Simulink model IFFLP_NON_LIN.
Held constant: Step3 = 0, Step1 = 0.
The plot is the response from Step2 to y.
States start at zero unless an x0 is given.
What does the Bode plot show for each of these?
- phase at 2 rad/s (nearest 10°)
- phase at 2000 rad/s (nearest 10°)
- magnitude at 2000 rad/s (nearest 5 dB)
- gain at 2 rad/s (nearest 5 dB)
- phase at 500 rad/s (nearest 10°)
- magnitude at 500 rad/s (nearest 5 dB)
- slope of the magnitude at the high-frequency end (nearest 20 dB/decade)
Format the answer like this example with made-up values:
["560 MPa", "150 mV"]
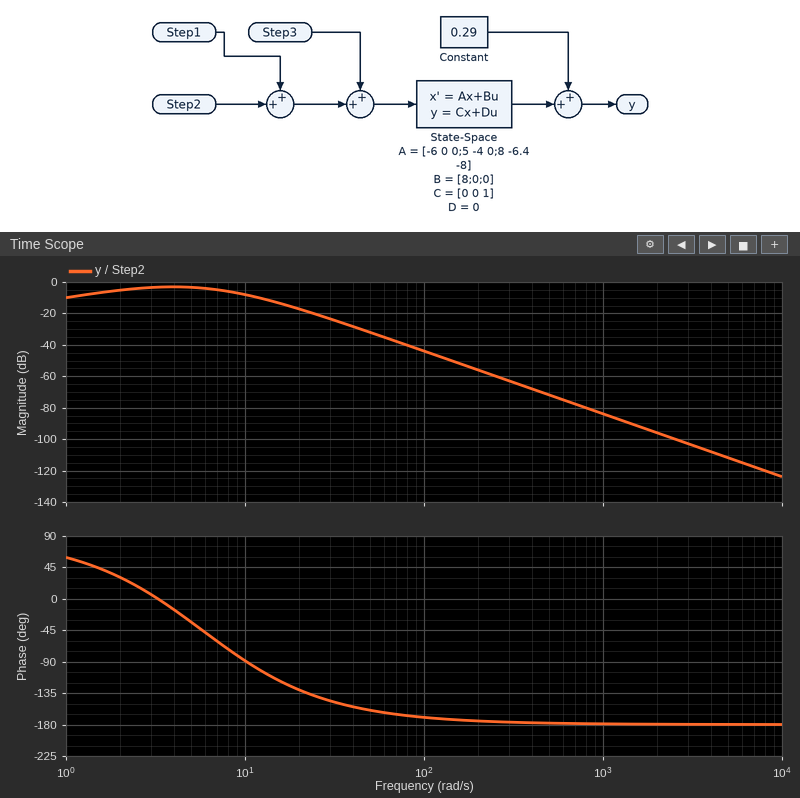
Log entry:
["30°", "-180°", "-95 dB", "-5 dB", "-180°", "-70 dB", "-40 dB/decade"]
